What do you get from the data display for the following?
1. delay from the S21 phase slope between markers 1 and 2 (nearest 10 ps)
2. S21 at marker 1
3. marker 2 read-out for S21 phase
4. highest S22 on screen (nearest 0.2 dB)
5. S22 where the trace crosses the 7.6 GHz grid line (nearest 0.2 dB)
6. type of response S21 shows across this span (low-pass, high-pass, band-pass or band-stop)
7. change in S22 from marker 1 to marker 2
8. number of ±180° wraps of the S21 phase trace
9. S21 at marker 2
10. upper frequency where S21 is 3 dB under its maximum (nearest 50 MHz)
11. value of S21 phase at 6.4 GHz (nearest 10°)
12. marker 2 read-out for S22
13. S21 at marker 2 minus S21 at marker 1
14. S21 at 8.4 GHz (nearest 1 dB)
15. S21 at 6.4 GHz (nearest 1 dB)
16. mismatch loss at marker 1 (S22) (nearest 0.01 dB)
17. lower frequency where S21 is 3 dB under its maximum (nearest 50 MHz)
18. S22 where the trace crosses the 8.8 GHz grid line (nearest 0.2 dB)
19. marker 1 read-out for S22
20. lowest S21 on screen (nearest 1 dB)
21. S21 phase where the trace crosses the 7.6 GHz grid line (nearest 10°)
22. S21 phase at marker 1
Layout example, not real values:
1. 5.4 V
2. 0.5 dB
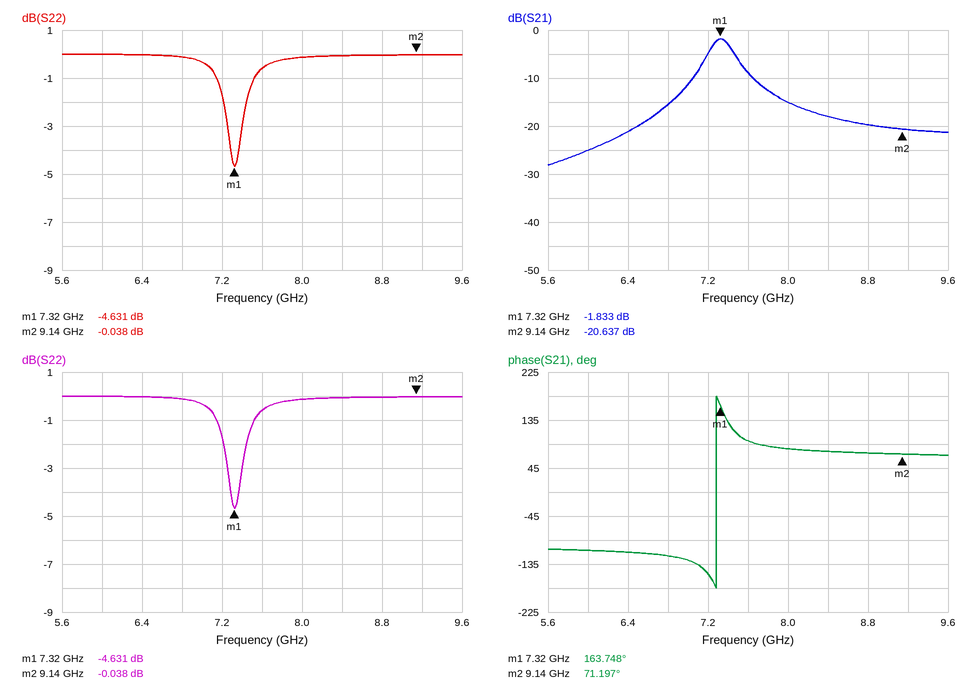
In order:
1. 140 ps
2. -1.833 dB
3. 71.197°
4. 0.0 dB
5. -0.6 dB
6. band-pass
7. 4.593 dB
8. 1
9. -20.637 dB
10. 7.45 GHz
11. -110°
12. -0.038 dB
13. -18.804 dB
14. -18 dB
15. -21 dB
16. 1.83 dB
17. 7.20 GHz
18. 0.0 dB
19. -4.631 dB
20. -28 dB
21. 100°
22. 163.748°
